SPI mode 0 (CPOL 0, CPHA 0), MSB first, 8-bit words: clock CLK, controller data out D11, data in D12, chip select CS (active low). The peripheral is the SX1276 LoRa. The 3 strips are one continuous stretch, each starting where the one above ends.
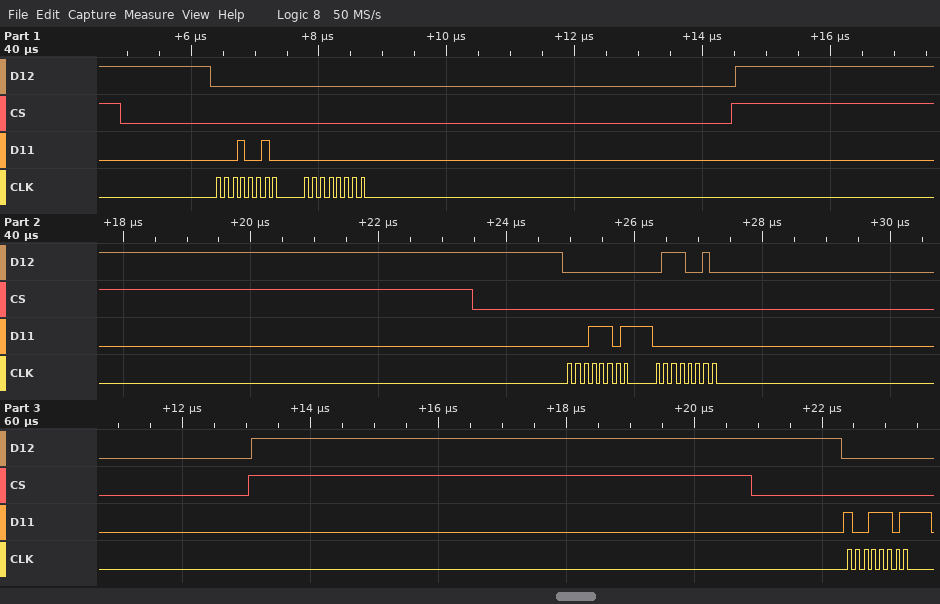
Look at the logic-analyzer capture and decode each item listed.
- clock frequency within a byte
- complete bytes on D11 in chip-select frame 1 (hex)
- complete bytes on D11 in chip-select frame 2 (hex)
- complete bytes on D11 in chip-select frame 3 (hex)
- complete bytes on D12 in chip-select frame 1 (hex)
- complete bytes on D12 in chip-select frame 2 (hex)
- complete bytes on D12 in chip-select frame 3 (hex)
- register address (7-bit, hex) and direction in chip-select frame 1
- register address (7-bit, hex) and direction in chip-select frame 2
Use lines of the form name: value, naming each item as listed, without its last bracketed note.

clock frequency within a byte: 8 MHz
complete bytes on D11 in chip-select frame 1: 12 00
complete bytes on D11 in chip-select frame 2: 1D 00
complete bytes on D11 in chip-select frame 3: 9D
complete bytes on D12 in chip-select frame 1: 00 00
complete bytes on D12 in chip-select frame 2: 00 72
complete bytes on D12 in chip-select frame 3: 00
register address (7-bit, hex) and direction in chip-select frame 1: 0x12 read
register address (7-bit, hex) and direction in chip-select frame 2: 0x1D read
